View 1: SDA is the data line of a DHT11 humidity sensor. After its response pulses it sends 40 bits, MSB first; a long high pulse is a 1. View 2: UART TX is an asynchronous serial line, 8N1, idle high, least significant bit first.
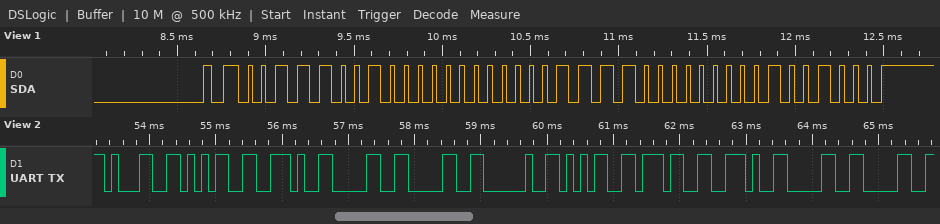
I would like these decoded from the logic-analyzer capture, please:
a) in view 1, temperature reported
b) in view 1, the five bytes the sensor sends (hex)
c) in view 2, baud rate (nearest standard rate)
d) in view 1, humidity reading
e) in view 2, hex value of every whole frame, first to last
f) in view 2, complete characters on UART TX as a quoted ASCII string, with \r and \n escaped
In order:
15.0 °C
39 00 0F 00 48
9600 baud
57 %
31 35 2E 30 30 20 35 37 2E 30 30
"15.00 57.00"
